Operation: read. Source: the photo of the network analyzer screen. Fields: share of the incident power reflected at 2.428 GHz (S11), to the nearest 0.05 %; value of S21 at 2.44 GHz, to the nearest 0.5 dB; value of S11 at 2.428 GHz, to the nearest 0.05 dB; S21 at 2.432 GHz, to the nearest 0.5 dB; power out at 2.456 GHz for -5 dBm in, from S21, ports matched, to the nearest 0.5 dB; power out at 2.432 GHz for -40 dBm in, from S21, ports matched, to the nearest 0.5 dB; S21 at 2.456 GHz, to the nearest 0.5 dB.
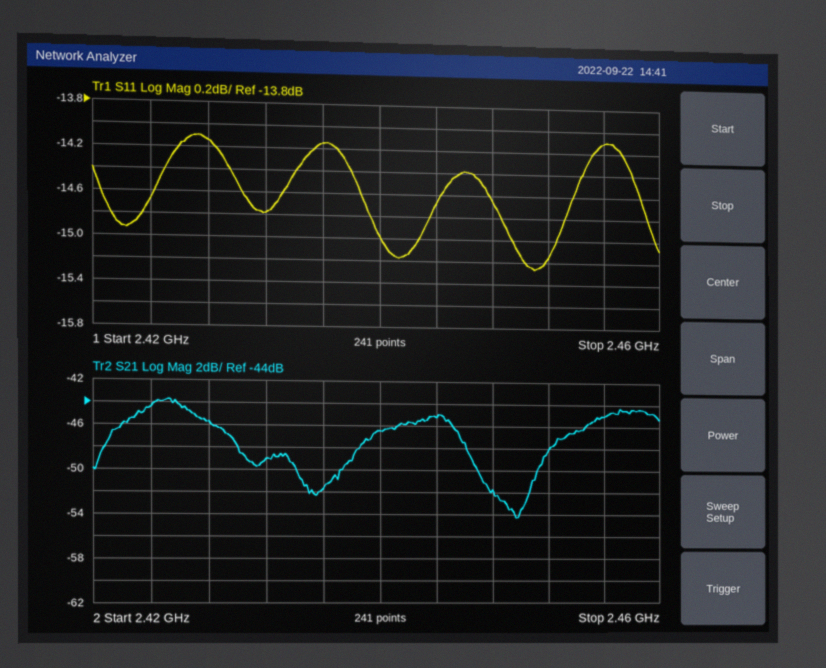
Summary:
3.85 %
-46.5 dB
-14.15 dB
-49.0 dB
-50.0 dBm
-89.0 dBm
-45.0 dB
